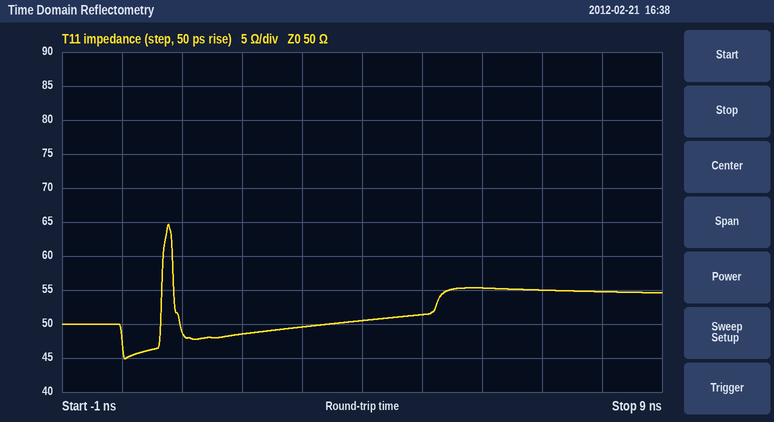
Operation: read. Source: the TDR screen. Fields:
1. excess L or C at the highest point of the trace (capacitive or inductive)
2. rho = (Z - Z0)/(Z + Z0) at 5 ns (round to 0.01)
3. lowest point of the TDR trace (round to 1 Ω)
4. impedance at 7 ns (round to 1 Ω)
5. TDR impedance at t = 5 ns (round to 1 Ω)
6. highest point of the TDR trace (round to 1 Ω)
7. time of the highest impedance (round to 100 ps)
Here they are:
inductive
+0.01
45 Ω
55 Ω
51 Ω
65 Ω
800 ps
